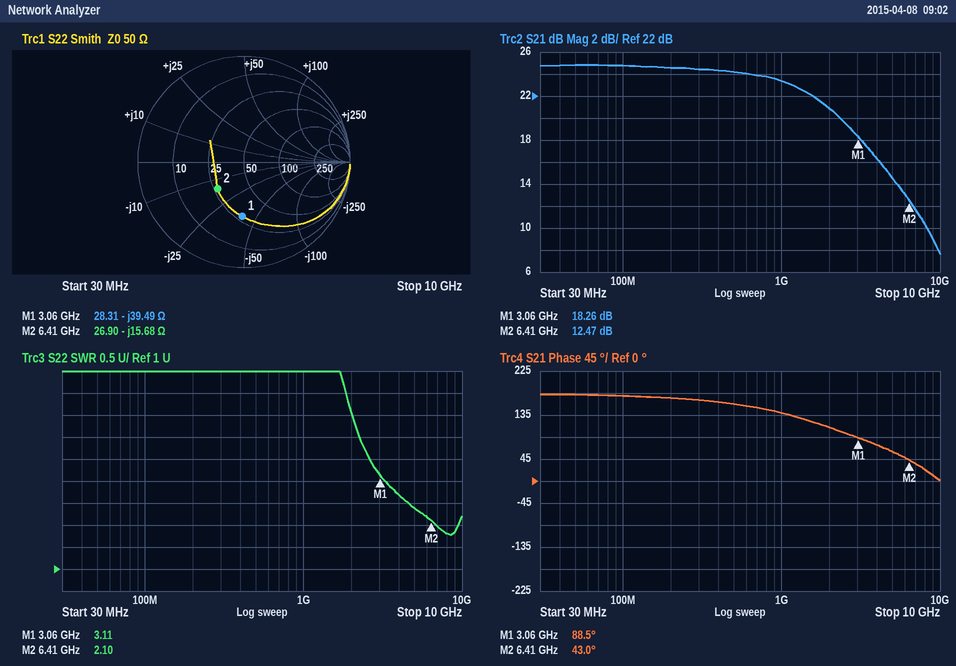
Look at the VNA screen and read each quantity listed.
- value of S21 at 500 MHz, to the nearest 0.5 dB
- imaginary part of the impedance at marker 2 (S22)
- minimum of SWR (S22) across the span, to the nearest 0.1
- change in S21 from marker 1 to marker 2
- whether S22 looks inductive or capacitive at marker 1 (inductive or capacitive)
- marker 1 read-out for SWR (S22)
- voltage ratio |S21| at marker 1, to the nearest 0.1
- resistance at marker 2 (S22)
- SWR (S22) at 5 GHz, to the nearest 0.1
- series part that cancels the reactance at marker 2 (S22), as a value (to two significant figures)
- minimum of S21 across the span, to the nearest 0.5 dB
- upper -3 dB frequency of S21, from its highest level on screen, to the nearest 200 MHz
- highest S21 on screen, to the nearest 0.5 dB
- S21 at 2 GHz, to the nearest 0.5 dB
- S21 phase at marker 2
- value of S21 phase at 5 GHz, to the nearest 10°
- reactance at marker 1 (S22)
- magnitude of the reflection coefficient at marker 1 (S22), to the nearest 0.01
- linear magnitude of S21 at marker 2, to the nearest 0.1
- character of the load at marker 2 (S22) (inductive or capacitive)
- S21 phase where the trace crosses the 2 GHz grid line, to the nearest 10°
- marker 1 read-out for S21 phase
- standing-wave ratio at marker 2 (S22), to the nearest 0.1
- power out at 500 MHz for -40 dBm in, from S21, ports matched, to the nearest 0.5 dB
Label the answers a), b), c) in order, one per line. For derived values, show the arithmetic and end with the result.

a) 24.0 dB
b) -15.68 Ω
c) 1.8
d) 12.47 − (18.26) = -5.79 dB
e) capacitive
f) 3.11
g) 10^(18.26/20) ≈ 8.2
h) 26.90 Ω
i) 2.4
j) L = 15.68 Ω/(2π × 6.41 GHz) ≈ 389 pH, so 390 pH to two significant figures
k) 7.5 dB
l) 1.6 GHz
m) 25.0 dB
n) 21.0 dB
o) 43.0°
p) 60°
q) -39.49 Ω
r) 0.51
s) 10^(12.47/20) ≈ 4.2
t) capacitive
u) 110°
v) 88.5°
w) 2.1
x) -40 dBm + (24.0 dB) = -16.0 dBm
